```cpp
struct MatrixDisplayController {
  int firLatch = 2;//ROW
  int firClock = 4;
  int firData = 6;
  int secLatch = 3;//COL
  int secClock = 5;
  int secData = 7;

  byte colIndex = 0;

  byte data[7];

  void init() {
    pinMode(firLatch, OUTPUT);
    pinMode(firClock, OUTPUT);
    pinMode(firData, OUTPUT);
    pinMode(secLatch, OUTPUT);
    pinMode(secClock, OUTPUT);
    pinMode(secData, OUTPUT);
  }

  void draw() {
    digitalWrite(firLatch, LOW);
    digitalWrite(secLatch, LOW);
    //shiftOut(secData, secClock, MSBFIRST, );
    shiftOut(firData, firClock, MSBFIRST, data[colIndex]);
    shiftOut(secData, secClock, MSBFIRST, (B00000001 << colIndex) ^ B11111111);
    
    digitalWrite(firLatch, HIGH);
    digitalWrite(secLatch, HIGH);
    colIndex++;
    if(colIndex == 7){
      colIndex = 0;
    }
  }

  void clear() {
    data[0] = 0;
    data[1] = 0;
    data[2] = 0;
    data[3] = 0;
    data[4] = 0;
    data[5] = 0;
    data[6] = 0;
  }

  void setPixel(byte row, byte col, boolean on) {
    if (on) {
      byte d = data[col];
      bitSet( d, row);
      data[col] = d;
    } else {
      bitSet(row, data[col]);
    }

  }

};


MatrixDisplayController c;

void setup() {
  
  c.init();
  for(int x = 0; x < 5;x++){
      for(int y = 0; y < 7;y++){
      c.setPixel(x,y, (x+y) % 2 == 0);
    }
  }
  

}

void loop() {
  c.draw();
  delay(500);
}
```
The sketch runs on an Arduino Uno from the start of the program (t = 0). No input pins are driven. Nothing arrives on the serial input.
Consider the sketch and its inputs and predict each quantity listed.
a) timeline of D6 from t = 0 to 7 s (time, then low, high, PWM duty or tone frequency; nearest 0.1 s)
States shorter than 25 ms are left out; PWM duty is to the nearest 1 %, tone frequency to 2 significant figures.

0 s high; 0.5 s low; 1 s high; 1.5 s low; 2 s high; 2.5 s low; 3 s high; 4 s low; 4.5 s high; 5 s low; 5.5 s high; 6 s low; 6.5 s high
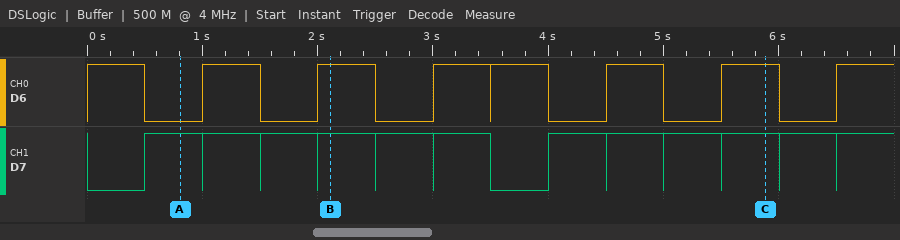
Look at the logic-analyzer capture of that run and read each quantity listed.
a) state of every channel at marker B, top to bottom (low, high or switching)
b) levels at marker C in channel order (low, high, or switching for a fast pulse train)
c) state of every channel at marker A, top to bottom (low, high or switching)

D6 high, D7 high
D6 high, D7 high
D6 low, D7 high
